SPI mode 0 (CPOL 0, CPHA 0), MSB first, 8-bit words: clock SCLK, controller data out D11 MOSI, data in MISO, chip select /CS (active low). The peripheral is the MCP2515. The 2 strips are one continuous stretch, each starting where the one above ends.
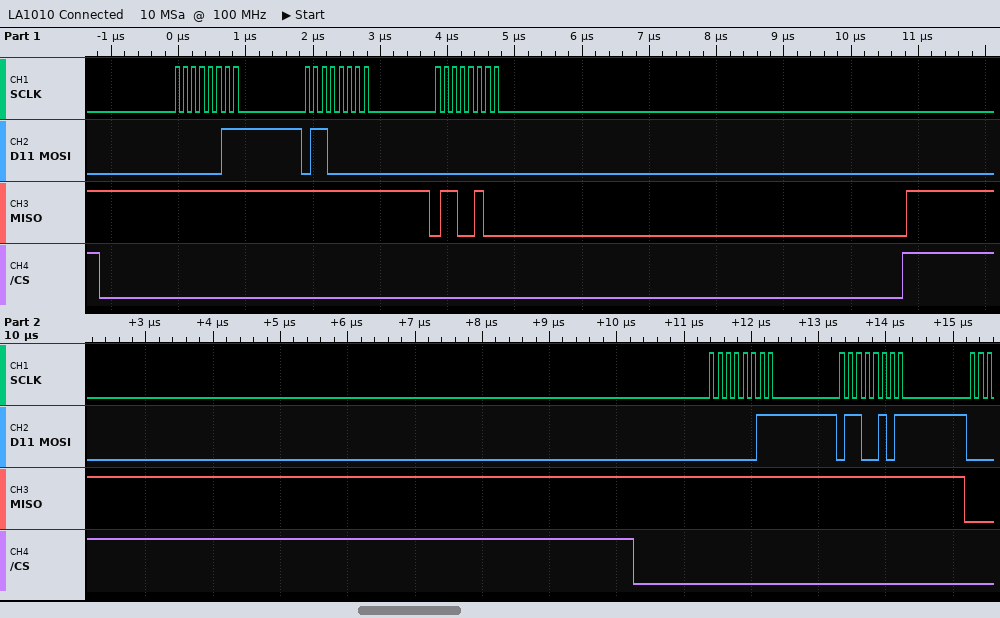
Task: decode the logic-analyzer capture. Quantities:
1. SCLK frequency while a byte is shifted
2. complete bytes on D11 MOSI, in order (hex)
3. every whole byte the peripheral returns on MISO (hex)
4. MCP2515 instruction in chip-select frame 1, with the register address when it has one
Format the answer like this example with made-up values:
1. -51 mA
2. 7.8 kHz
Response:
1. 8 MHz
2. 03 60 00 03 65
3. FF FF 64 FF FF
4. READ 0x60
